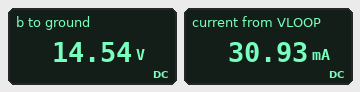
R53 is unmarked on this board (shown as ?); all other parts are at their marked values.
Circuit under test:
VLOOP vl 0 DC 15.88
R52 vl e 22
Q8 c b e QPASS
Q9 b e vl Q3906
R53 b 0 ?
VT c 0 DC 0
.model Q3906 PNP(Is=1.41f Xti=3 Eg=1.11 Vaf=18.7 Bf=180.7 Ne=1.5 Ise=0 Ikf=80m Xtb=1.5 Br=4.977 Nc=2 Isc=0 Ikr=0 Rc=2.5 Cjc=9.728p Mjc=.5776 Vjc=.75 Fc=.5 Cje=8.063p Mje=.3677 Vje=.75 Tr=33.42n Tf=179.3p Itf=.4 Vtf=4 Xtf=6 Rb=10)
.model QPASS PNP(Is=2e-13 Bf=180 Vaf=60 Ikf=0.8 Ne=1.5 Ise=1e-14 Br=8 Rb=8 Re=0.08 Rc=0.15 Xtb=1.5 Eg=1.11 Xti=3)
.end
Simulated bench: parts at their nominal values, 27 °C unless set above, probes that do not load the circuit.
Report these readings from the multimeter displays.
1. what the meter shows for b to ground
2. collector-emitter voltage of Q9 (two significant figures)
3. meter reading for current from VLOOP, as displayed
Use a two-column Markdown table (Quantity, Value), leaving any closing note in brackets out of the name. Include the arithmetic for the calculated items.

| Quantity | Value |
|---|---|
| what the meter shows for b to ground | 14.54 V |
| collector-emitter voltage of Q9 | 14.54 V - 15.88 V = -1.3 V |
| meter reading for current from VLOOP, as displayed | 30.93 mA |
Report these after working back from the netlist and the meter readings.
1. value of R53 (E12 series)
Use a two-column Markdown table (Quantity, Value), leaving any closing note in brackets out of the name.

| Quantity | Value |
|---|---|
| value of R53 | 33 kΩ |
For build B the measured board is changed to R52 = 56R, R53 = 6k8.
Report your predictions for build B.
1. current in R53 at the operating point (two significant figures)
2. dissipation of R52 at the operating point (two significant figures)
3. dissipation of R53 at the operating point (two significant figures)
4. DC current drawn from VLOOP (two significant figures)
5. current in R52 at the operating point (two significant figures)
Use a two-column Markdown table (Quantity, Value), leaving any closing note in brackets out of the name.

| Quantity | Value |
|---|---|
| current in R53 at the operating point | 2.1 mA |
| dissipation of R52 at the operating point | 9.4 mW |
| dissipation of R53 at the operating point | 31 mW |
| DC current drawn from VLOOP | 15 mA |
| current in R52 at the operating point | 13 mA |
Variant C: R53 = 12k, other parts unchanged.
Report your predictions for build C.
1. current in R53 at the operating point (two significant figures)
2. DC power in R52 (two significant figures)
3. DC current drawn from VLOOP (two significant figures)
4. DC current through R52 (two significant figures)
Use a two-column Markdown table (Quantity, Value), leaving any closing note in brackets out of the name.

| Quantity | Value |
|---|---|
| current in R53 at the operating point | 1.2 mA |
| DC power in R52 | 23 mW |
| DC current drawn from VLOOP | 33 mA |
| DC current through R52 | 32 mA |
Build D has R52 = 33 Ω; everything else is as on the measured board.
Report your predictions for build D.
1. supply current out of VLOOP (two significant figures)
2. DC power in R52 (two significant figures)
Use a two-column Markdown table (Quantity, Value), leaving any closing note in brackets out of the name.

| Quantity | Value |
|---|---|
| supply current out of VLOOP | 21 mA |
| DC power in R52 | 14 mW |
